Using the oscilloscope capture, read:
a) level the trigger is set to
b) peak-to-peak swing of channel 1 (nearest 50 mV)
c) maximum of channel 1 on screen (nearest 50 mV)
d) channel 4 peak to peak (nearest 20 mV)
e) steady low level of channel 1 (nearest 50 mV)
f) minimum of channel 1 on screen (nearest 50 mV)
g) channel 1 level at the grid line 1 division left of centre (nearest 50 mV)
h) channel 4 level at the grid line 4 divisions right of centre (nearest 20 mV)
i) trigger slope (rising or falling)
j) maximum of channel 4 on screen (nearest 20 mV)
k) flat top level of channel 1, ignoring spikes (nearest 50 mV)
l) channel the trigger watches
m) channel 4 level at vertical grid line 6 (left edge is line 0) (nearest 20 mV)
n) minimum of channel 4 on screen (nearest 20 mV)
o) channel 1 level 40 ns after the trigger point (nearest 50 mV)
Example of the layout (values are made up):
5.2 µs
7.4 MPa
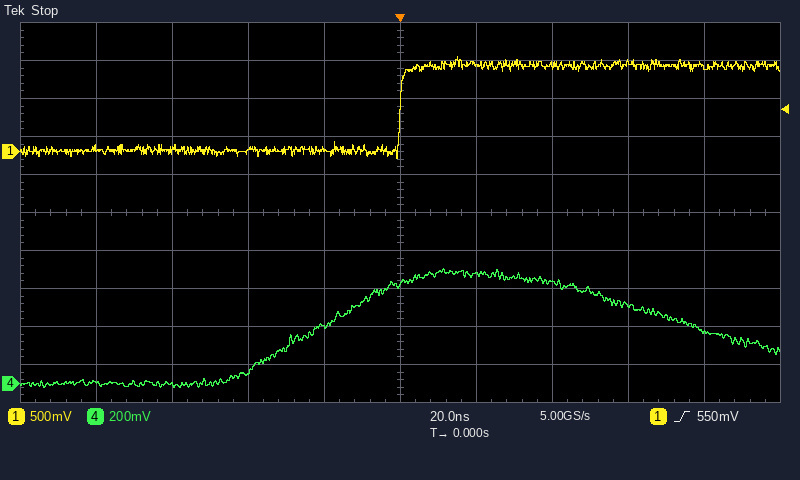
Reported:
550 mV
1.35 V
1.25 V
620 mV
0 mV
-100 mV
50 mV
280 mV
rising
600 mV
1.15 V
channel 1
580 mV
-20 mV
1.15 V
